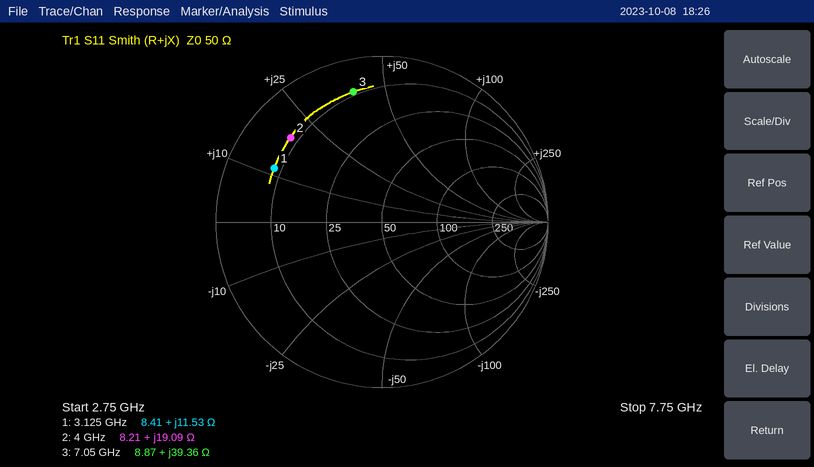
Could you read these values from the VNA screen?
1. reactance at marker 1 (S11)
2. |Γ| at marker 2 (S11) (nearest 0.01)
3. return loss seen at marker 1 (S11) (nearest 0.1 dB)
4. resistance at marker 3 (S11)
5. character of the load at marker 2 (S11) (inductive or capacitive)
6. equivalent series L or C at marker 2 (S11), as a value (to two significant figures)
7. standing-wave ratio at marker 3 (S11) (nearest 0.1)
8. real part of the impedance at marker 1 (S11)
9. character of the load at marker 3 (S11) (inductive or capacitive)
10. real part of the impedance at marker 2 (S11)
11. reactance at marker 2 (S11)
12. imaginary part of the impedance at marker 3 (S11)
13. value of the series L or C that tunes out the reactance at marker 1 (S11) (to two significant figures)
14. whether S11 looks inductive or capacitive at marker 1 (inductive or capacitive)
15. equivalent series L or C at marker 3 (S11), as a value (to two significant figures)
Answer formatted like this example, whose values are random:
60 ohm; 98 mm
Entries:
+11.53 Ω; 0.75; 2.8 dB; 8.87 Ω; inductive; 760 pH; 9.2; 8.41 Ω; inductive; 8.21 Ω; +19.09 Ω; +39.36 Ω; 4.4 pF; inductive; 890 pH
